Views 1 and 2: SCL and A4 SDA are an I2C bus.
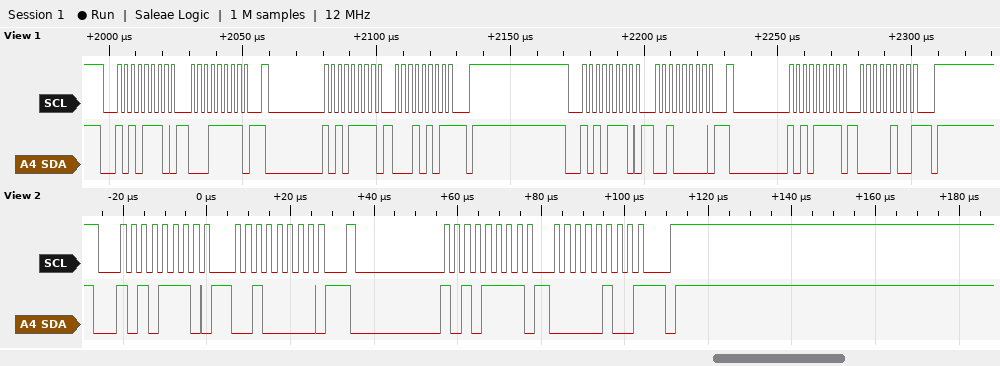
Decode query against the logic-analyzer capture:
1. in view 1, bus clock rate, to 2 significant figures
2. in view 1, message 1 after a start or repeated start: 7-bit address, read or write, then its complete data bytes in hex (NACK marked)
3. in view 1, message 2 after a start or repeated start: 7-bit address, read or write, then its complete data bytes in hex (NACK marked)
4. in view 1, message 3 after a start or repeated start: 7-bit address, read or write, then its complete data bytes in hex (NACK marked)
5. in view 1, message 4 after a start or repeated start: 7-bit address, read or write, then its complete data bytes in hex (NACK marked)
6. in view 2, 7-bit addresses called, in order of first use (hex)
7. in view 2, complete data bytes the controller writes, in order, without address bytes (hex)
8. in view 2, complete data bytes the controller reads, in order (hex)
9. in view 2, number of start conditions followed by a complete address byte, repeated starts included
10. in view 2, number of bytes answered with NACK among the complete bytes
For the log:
400 kHz
0x57 write: 1F
0x57 read: 15 NACK
0x57 write: 20
0x57 read: 04 NACK
0x57
20
04
2
1
